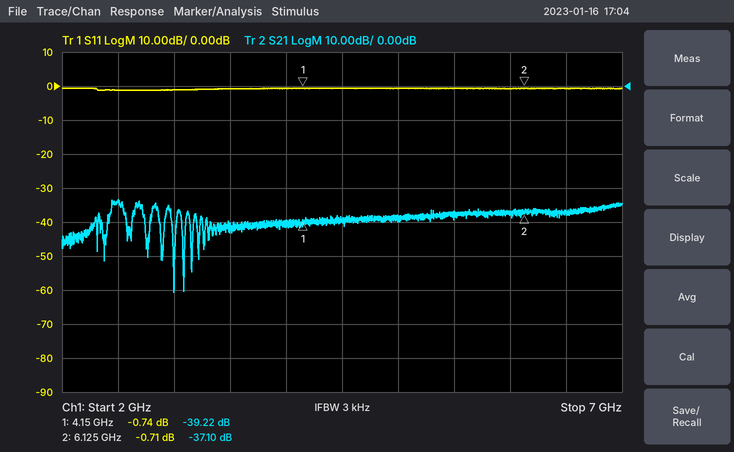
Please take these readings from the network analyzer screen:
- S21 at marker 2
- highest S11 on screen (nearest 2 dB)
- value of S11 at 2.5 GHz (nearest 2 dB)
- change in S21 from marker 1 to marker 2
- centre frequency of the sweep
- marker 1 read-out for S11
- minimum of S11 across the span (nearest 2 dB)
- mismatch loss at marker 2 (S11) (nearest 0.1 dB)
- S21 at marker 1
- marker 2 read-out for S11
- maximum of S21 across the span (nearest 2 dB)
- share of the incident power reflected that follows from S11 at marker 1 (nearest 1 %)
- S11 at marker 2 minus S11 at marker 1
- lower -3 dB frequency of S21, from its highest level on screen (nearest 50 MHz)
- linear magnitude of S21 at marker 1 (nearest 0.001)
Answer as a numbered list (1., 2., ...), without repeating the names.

1. -37.10 dB
2. 0 dB
3. -2 dB
4. 2.12 dB
5. 4.5 GHz
6. -0.74 dB
7. -2 dB
8. 8.2 dB
9. -39.22 dB
10. -0.71 dB
11. -34 dB
12. 84 %
13. 0.03 dB
14. 2.45 GHz
15. 0.011
